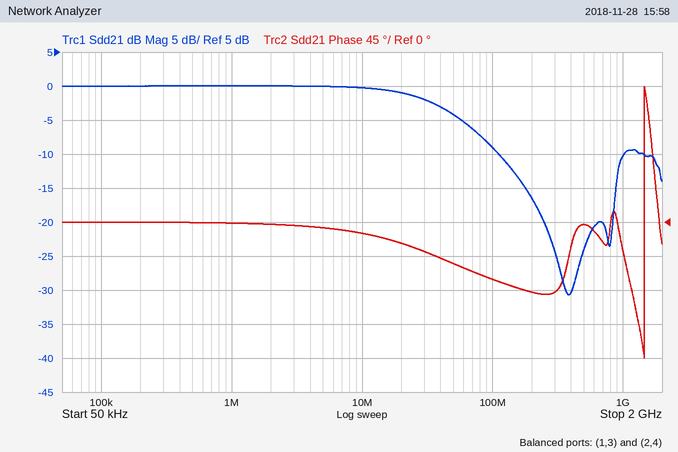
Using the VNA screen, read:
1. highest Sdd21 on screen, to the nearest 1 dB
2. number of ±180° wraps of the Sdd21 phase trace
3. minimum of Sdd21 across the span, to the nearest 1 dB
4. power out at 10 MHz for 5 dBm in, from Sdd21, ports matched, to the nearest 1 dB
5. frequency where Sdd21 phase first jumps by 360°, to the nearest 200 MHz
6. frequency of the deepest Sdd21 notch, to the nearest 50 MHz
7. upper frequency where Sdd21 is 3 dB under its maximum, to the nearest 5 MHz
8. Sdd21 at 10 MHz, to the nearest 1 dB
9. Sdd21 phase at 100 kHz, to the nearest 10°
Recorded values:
0 dB
1
-31 dB
5 dBm
1.4 GHz
400 MHz
40 MHz
0 dB
0°
